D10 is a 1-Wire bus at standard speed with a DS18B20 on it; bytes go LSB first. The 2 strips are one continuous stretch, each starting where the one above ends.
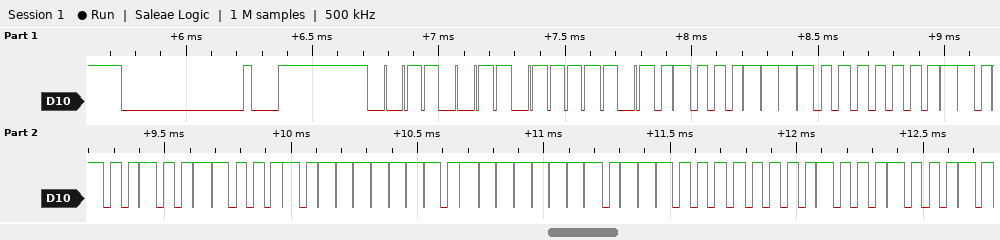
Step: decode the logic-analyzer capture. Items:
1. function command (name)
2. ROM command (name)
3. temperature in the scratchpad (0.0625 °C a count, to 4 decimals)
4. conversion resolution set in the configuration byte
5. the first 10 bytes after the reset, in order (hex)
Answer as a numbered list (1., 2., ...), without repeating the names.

1. Read Scratchpad
2. Skip ROM
3. 30.1250 °C
4. 12 bits
5. CC BE E2 01 4B 46 7F FF 0E 10
